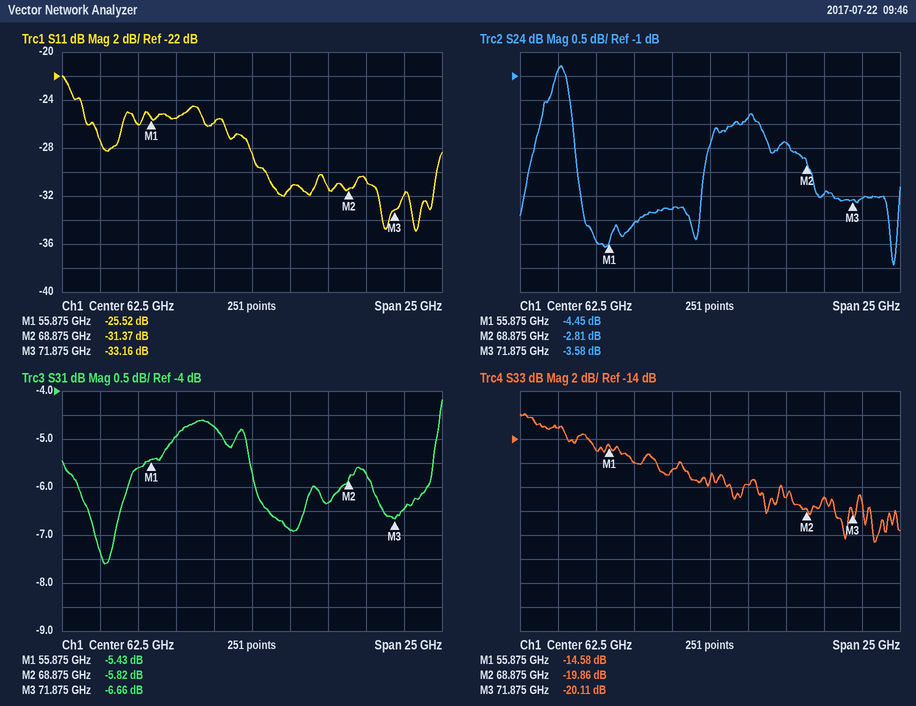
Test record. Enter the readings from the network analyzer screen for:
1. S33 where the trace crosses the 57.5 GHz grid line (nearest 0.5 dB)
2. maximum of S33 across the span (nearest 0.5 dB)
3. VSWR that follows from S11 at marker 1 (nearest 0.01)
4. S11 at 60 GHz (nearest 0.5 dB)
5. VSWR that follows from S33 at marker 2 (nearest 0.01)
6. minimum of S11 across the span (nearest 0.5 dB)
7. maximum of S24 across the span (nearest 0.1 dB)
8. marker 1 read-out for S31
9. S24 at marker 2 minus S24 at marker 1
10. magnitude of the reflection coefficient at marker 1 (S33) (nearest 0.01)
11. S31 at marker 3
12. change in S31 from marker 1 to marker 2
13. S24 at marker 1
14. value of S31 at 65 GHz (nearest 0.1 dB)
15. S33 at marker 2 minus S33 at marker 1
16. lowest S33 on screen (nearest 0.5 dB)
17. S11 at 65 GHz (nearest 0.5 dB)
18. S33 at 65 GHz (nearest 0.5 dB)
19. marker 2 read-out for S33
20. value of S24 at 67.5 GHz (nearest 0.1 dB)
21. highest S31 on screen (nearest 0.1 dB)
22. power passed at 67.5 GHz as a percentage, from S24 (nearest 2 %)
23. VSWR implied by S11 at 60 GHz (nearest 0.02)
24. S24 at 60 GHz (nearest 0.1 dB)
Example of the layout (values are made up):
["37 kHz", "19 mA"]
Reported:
["-16.0 dB", "-12.0 dB", "1.11", "-26.0 dB", "1.23", "-35.0 dB", "-0.8 dB", "-5.43 dB", "1.64 dB", "0.19", "-6.66 dB", "-0.39 dB", "-4.45 dB", "-6.9 dB", "-5.28 dB", "-22.5 dB", "-31.5 dB", "-18.0 dB", "-19.86 dB", "-2.4 dB", "-4.2 dB", "58 %", "1.10", "-3.8 dB"]
